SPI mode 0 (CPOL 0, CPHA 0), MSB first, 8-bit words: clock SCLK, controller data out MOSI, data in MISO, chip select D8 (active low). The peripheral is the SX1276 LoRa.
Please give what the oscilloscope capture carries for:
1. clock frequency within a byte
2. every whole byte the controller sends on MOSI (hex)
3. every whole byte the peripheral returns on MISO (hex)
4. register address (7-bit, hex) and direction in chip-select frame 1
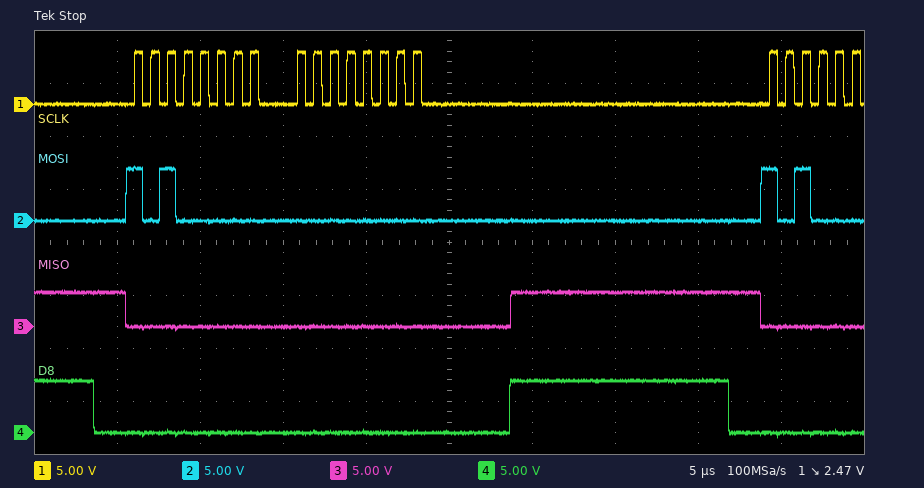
1 MHz
A0 00
00 00
0x20 write
